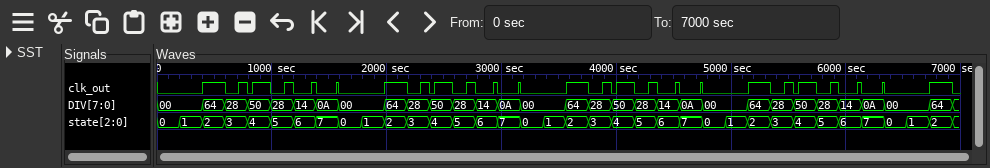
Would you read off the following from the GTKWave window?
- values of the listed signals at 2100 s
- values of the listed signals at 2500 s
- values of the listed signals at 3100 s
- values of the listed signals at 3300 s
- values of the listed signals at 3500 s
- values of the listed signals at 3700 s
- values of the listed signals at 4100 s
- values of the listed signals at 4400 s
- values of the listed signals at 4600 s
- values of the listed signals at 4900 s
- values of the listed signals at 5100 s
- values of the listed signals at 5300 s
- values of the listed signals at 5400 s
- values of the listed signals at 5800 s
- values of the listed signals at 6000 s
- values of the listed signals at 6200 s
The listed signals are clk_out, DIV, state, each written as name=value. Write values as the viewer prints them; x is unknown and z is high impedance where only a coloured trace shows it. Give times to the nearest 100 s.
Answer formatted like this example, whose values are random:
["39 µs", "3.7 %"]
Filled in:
["clk_out=1, DIV=64, state=2", "clk_out=1, DIV=50, state=4", "clk_out=0, DIV=0A, state=7", "clk_out=0, DIV=00, state=0", "clk_out=0, DIV=00, state=1", "clk_out=1, DIV=64, state=2", "clk_out=1, DIV=50, state=4", "clk_out=0, DIV=14, state=6", "clk_out=0, DIV=0A, state=7", "clk_out=0, DIV=00, state=0", "clk_out=0, DIV=00, state=1", "clk_out=1, DIV=64, state=2", "clk_out=0, DIV=28, state=3", "clk_out=0, DIV=28, state=5", "clk_out=0, DIV=14, state=6", "clk_out=0, DIV=0A, state=7"]
